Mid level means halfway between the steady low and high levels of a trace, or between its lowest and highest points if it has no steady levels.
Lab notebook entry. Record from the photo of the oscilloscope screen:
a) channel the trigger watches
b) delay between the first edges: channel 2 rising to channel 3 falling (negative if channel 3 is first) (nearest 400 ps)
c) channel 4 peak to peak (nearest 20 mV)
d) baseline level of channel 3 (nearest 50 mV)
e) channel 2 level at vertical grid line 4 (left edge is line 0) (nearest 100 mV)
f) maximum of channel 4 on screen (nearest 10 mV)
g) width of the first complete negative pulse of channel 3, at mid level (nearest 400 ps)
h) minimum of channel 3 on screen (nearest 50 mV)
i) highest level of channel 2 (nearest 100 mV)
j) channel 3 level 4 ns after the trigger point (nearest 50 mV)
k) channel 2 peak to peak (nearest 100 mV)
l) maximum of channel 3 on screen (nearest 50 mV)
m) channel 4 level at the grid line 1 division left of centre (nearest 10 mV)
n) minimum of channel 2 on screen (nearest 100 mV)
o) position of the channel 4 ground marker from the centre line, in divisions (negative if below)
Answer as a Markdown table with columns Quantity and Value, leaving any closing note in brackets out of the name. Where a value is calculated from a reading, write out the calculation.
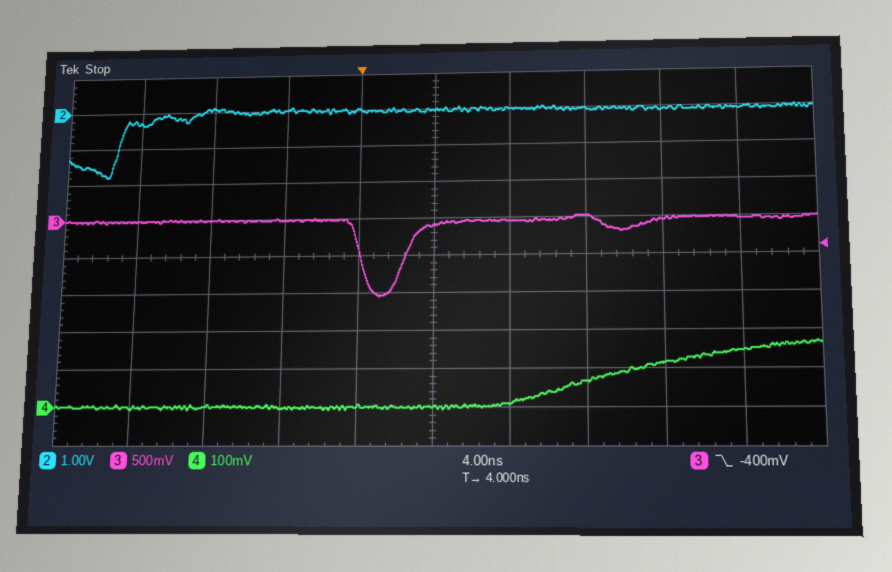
| Quantity | Value |
|---|---|
| channel the trigger watches | channel 3 |
| delay between the first edges: channel 2 rising to channel 3 falling (negative if channel 3 is first) | +13.2 ns |
| channel 4 peak to peak | 180 mV |
| baseline level of channel 3 | 0 mV |
| channel 2 level at vertical grid line 4 (left edge is line 0) | 0.0 V |
| maximum of channel 4 on screen | 170 mV |
| width of the first complete negative pulse of channel 3, at mid level | 2.4 ns |
| minimum of channel 3 on screen | -1.05 V |
| highest level of channel 2 | 100 mV |
| channel 3 level 4 ns after the trigger point | -100 mV |
| channel 2 peak to peak | 100 mV − (-1.8 V) = 1.9 V |
| maximum of channel 3 on screen | 50 mV |
| channel 4 level at the grid line 1 division left of centre | 0 mV |
| minimum of channel 2 on screen | -1.8 V |
| position of the channel 4 ground marker from the centre line, in divisions | -4.0 div |
